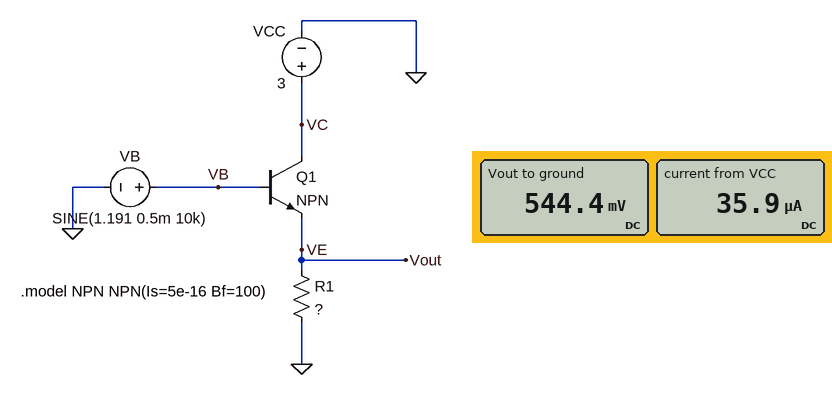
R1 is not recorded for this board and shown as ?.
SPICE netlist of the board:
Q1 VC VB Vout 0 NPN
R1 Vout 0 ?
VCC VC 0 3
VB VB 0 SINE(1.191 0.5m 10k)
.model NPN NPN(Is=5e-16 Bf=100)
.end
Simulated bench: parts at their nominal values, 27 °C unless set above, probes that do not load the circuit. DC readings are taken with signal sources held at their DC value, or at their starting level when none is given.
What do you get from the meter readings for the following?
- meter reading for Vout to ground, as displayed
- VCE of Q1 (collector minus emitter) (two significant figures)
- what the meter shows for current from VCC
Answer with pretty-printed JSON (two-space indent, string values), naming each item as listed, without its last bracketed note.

{
  "meter reading for Vout to ground, as displayed": "544.4 mV",
  "VCE of Q1 (collector minus emitter)": "2.5 V",
  "what the meter shows for current from VCC": "35.9 µA"
}
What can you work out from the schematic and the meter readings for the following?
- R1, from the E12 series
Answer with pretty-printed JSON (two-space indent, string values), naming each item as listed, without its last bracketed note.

{
  "R1, from the E12 series": "15 kΩ"
}
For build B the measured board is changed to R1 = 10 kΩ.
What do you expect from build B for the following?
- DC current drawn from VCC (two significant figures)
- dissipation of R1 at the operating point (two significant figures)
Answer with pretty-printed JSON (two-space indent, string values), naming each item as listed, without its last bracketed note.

{
  "DC current drawn from VCC": "53 µA",
  "dissipation of R1 at the operating point": "29 µW"
}
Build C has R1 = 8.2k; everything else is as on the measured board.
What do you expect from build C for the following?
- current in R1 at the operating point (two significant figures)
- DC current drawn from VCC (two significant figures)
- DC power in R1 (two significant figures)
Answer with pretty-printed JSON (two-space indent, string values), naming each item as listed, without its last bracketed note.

{
  "current in R1 at the operating point": "65 µA",
  "DC current drawn from VCC": "64 µA",
  "DC power in R1": "34 µW"
}
